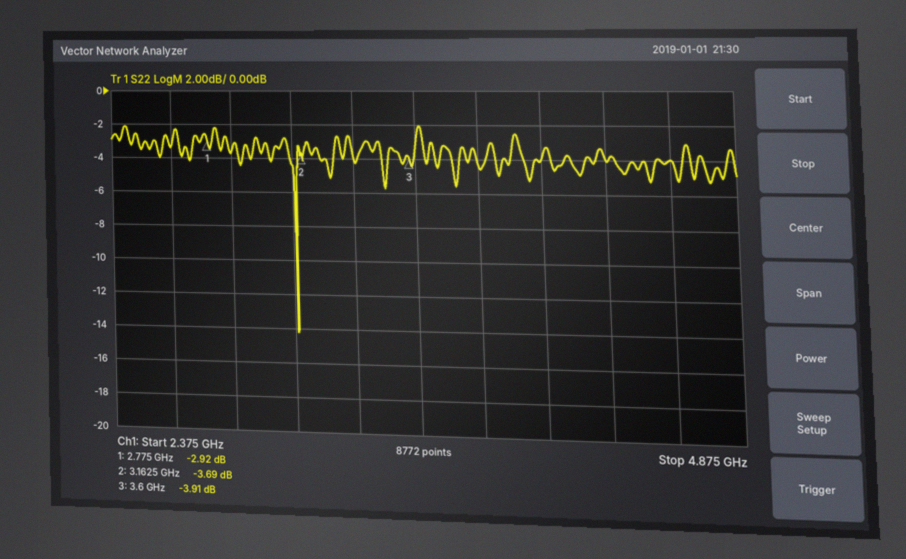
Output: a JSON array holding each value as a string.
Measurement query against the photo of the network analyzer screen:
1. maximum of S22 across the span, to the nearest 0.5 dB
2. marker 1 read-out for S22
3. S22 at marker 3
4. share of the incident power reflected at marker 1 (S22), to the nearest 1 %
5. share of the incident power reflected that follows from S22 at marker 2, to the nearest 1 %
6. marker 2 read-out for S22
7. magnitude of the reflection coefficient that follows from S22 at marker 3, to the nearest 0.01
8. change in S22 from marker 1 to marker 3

["-2.0 dB", "-2.92 dB", "-3.91 dB", "51 %", "43 %", "-3.69 dB", "0.64", "-0.99 dB"]
